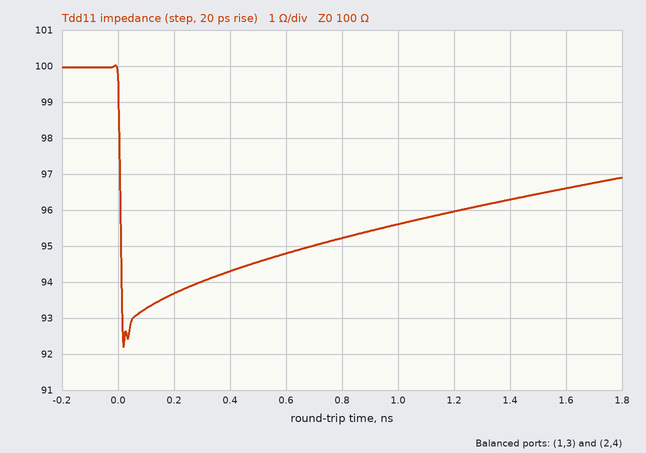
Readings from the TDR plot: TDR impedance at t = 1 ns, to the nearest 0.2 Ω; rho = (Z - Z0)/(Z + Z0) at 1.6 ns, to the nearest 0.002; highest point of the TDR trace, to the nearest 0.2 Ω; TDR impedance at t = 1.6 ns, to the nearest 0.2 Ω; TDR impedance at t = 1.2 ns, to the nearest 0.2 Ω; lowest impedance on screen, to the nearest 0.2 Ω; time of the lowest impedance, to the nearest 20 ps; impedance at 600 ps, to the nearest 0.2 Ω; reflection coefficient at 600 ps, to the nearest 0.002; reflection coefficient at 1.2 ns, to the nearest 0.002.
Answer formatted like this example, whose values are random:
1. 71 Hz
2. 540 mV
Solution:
1. 95.6 Ω
2. -0.018
3. 100.0 Ω
4. 96.6 Ω
5. 96.0 Ω
6. 92.2 Ω
7. 20 ps
8. 94.8 Ω
9. -0.026
10. -0.020
